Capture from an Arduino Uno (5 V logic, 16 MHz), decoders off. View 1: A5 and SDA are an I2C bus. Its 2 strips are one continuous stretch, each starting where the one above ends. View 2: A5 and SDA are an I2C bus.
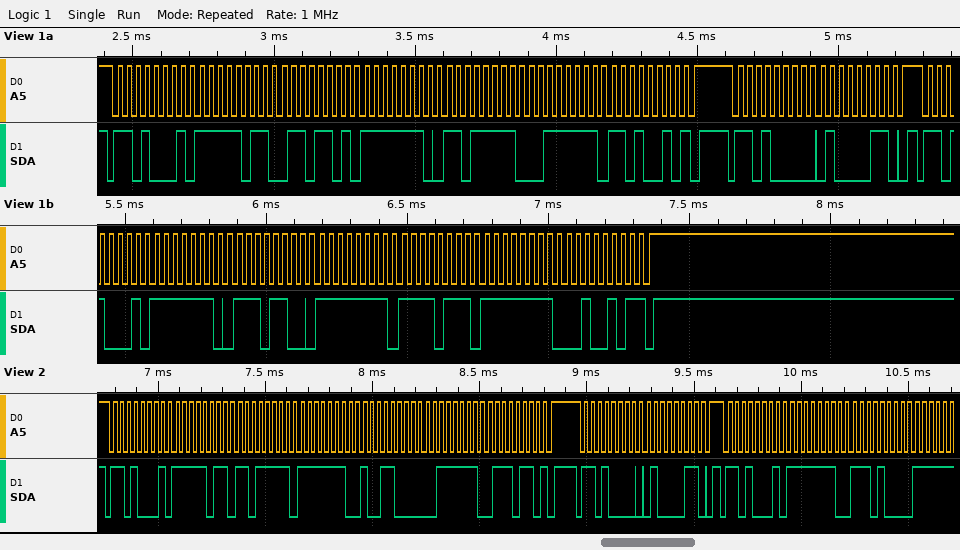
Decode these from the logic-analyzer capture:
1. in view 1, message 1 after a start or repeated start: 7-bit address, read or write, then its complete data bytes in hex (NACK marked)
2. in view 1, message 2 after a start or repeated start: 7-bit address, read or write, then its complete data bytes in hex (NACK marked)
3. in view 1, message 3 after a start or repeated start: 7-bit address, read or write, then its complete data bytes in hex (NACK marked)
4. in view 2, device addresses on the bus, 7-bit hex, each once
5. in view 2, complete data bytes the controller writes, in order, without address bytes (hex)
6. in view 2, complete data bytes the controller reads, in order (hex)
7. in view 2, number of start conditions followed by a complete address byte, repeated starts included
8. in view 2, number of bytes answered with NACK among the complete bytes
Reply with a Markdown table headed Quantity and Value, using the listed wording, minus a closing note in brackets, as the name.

| Quantity | Value |
|---|---|
| in view 1, message 1 after a start or repeated start: 7-bit address, read or write, then its complete data bytes in hex | 0x68 read: FB 6D FE DF 3F D2 NACK |
| in view 1, message 2 after a start or repeated start: 7-bit address, read or write, then its complete data bytes in hex | 0x68 write: 43 |
| in view 1, message 3 after a start or repeated start: 7-bit address, read or write, then its complete data bytes in hex | 0x68 read: FE EC FF F7 FF 25 NACK |
| in view 2, device addresses on the bus, 7-bit hex, each once | 0x68 |
| in view 2, complete data bytes the controller writes, in order, without address bytes | 43 |
| in view 2, complete data bytes the controller reads, in order | FB DF FE 98 3F 76 FE E8 |
| in view 2, number of start conditions followed by a complete address byte, repeated starts included | 3 |
| in view 2, number of bytes answered with NACK among the complete bytes | 1 |
